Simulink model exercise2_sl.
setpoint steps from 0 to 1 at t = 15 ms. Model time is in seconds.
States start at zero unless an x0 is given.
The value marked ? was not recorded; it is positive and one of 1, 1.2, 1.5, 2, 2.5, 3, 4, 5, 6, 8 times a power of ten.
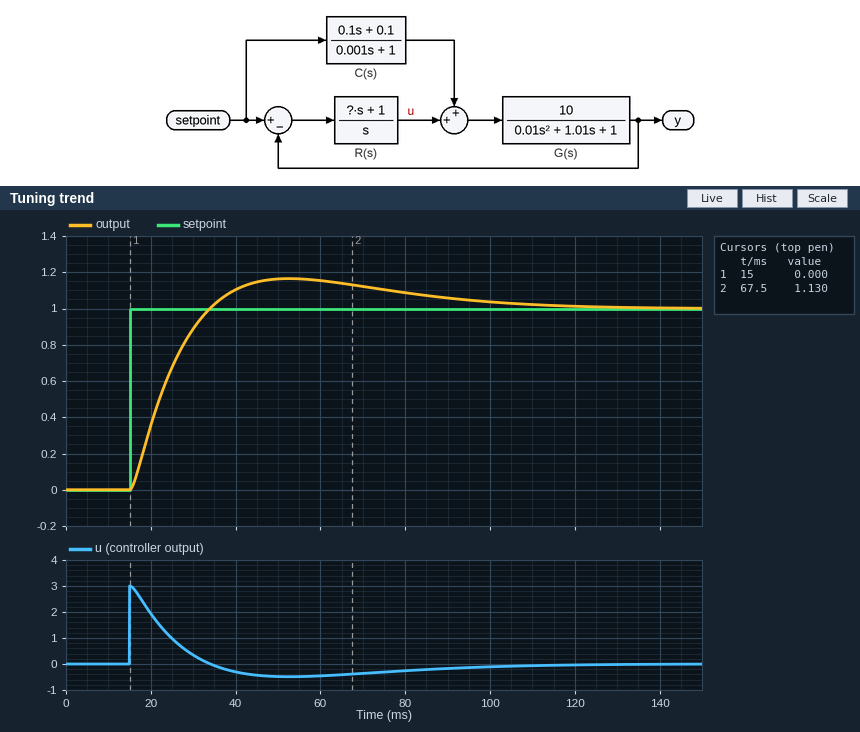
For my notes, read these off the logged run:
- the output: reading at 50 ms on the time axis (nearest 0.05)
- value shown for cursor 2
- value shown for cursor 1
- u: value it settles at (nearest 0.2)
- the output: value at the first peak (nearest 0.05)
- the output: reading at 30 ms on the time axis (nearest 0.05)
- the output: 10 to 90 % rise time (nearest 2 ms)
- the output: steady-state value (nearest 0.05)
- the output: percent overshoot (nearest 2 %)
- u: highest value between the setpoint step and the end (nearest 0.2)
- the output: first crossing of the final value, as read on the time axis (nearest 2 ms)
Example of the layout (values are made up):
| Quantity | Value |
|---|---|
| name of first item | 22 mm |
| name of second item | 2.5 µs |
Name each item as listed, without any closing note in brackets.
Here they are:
| Quantity | Value |
|---|---|
| the output: reading at 50 ms on the time axis | 1.15 |
| value shown for cursor 2 | 1.130 |
| value shown for cursor 1 | 0.000 |
| u: value it settles at | 0.0 |
| the output: value at the first peak | 1.15 |
| the output: reading at 30 ms on the time axis | 0.90 |
| the output: 10 to 90 % rise time | 14 ms |
| the output: steady-state value | 1.00 |
| the output: percent overshoot | 16 % |
| u: highest value between the setpoint step and the end | 3.0 |
| the output: first crossing of the final value, as read on the time axis | 34 ms |
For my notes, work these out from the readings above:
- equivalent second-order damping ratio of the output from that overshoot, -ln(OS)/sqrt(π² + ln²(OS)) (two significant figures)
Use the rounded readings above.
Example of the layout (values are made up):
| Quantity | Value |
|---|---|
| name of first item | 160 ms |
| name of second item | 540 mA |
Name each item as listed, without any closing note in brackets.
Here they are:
| Quantity | Value |
|---|---|
| equivalent second-order damping ratio of the output from that overshoot, -ln(OS)/sqrt(π² + ln²(OS)) | 0.50 |
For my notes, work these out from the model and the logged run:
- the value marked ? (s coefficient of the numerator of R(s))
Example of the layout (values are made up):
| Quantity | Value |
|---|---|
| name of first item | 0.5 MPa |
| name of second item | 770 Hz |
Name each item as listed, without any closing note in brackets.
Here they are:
| Quantity | Value |
|---|---|
| the value marked ? (s coefficient of the numerator of R(s)) | 3 |
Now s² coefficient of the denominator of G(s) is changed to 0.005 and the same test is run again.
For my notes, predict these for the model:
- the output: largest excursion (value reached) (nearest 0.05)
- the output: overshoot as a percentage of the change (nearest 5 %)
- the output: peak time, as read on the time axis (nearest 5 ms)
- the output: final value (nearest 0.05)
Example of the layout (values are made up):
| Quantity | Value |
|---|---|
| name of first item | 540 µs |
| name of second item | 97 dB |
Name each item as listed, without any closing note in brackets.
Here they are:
| Quantity | Value |
|---|---|
| the output: largest excursion (value reached) | 1.10 |
| the output: overshoot as a percentage of the change | 10 % |
| the output: peak time, as read on the time axis | 40 ms |
| the output: final value | 1.00 |
